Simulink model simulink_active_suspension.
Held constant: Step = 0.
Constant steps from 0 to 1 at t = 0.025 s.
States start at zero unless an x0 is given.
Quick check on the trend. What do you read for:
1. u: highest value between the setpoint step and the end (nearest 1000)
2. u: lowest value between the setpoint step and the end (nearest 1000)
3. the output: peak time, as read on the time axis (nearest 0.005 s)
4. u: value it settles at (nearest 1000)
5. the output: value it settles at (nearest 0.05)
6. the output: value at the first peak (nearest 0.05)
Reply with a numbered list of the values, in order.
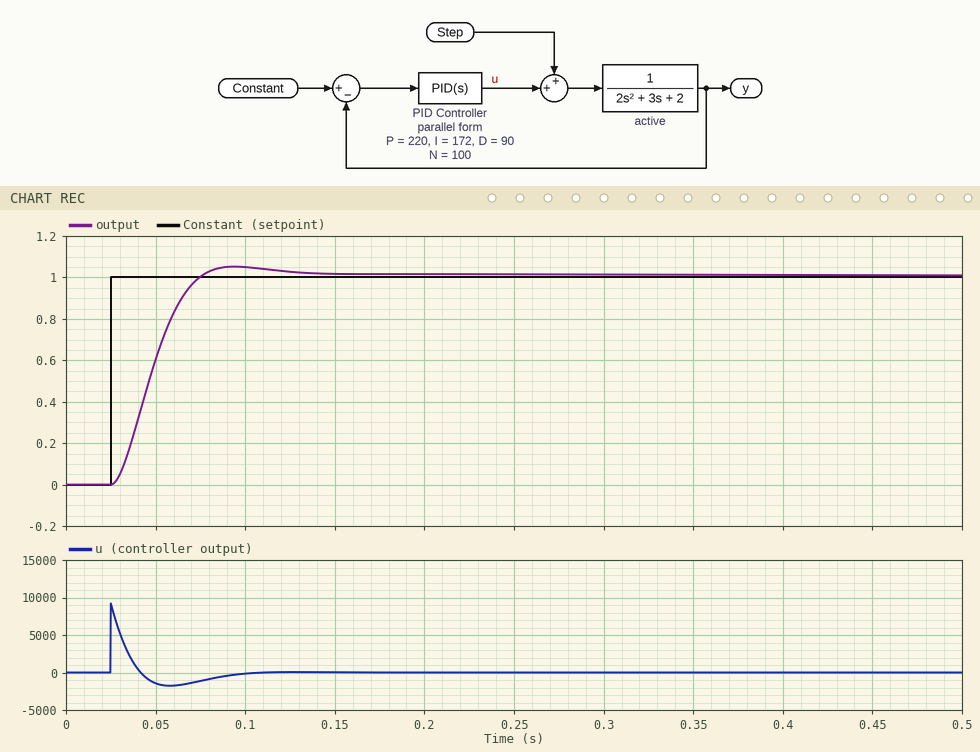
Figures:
1. 9000
2. -2000
3. 0.095 s
4. 0
5. 1.00
6. 1.05
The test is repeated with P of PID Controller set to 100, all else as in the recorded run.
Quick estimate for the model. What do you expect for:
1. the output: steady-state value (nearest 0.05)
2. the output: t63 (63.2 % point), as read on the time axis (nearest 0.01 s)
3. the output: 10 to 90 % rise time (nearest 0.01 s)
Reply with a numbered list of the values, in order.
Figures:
1. 1.00
2. 0.05 s
3. 0.03 s
